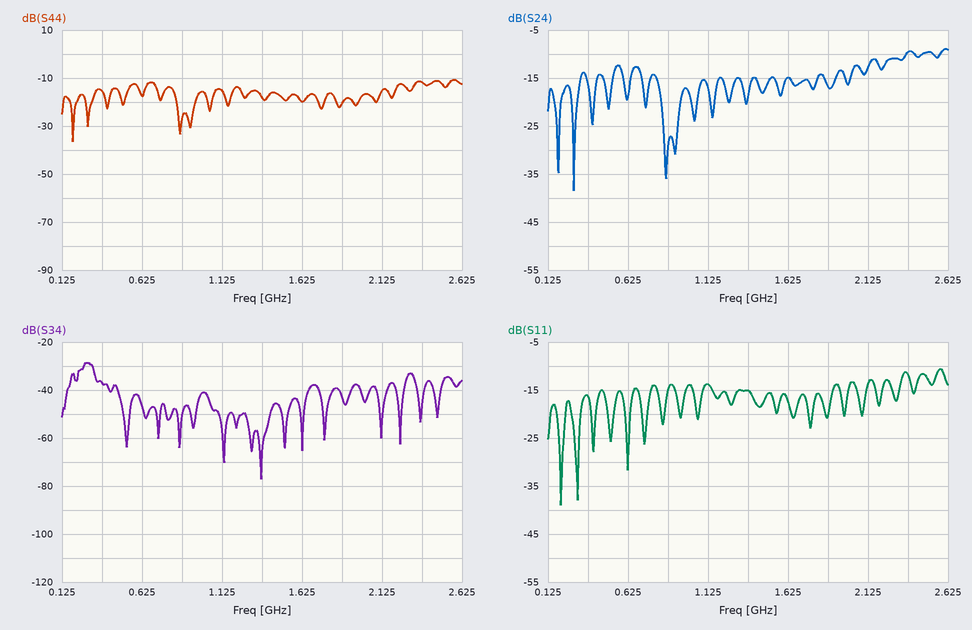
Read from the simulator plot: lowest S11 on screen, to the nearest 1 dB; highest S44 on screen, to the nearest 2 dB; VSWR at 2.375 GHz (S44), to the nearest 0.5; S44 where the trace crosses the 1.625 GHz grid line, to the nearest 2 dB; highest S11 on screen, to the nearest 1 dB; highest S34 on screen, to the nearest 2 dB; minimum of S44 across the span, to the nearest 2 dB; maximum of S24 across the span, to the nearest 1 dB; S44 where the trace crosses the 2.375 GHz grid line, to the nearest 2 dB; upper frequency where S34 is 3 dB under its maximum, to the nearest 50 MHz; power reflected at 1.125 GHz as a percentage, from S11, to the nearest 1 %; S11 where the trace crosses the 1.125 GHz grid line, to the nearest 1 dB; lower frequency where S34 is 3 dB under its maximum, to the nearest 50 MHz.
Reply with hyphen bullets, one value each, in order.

- -39 dB
- -10 dB
- 1.5
- -20 dB
- -11 dB
- -28 dB
- -36 dB
- -9 dB
- -12 dB
- 300 MHz
- 4 %
- -14 dB
- 250 MHz
